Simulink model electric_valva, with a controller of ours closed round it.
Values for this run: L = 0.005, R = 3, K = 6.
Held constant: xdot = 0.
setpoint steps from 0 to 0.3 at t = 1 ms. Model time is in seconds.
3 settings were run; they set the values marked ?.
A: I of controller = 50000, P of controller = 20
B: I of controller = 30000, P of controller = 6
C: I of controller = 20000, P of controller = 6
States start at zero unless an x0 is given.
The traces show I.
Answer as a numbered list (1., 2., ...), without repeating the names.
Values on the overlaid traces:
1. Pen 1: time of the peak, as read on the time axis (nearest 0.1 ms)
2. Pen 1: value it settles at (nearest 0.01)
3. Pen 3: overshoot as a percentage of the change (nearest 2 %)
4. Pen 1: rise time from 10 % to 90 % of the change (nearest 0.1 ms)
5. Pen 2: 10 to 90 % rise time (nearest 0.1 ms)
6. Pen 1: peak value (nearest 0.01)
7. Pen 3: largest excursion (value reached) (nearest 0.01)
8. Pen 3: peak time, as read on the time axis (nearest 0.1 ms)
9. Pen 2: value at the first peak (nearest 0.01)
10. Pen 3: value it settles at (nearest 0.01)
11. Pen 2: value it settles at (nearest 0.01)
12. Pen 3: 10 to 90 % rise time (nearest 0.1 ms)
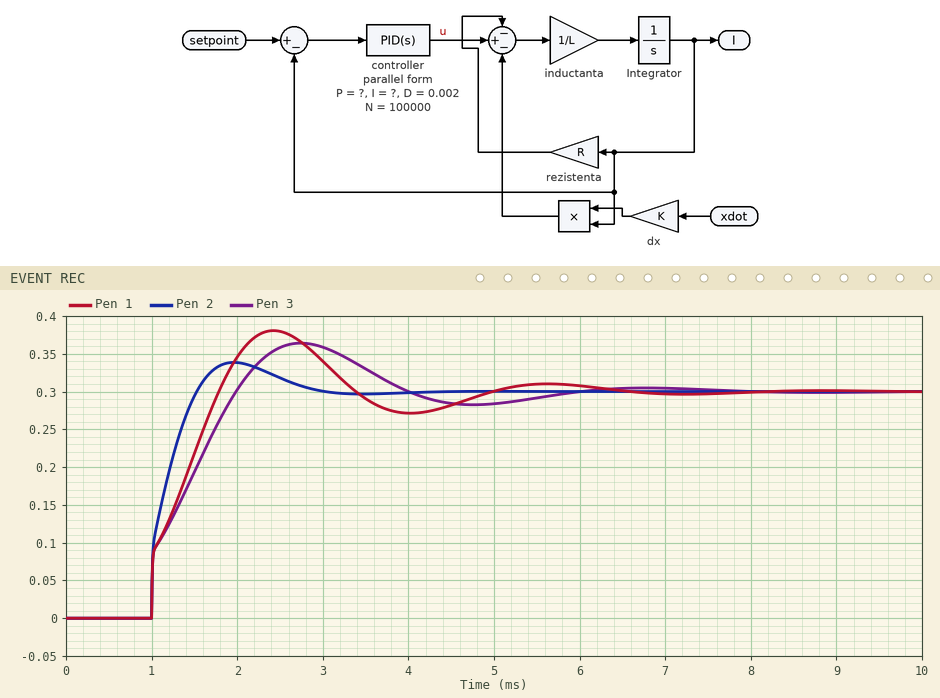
1. 2.4 ms
2. 0.30
3. 22 %
4. 0.7 ms
5. 0.4 ms
6. 0.38
7. 0.36
8. 2.7 ms
9. 0.34
10. 0.30
11. 0.30
12. 0.8 ms
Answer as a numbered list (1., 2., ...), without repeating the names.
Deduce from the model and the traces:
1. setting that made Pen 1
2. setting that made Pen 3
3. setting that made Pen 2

1. B
2. C
3. A
